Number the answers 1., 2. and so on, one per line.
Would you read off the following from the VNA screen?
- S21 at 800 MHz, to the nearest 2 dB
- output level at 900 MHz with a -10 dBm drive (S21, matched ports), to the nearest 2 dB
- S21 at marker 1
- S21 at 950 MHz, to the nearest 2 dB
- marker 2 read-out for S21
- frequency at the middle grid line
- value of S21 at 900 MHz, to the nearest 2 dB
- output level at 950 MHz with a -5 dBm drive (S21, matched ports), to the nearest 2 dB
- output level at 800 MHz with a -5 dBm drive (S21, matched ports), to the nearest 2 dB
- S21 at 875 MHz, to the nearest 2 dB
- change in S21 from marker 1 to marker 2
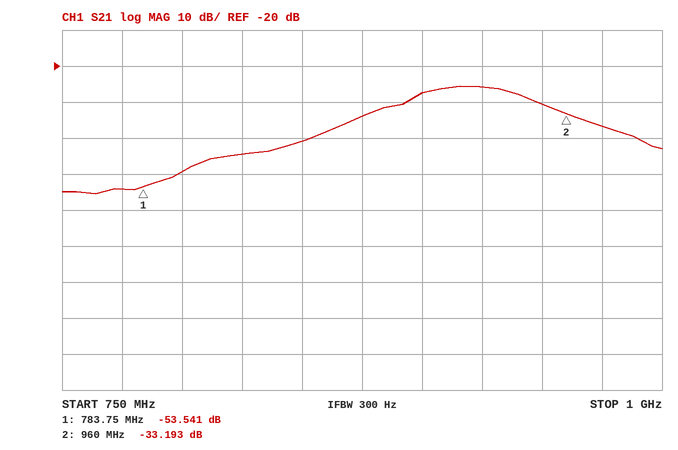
1. -50 dB
2. -38 dBm
3. -53.541 dB
4. -30 dB
5. -33.193 dB
6. 875 MHz
7. -28 dB
8. -36 dBm
9. -54 dBm
10. -34 dB
11. 20.348 dB
